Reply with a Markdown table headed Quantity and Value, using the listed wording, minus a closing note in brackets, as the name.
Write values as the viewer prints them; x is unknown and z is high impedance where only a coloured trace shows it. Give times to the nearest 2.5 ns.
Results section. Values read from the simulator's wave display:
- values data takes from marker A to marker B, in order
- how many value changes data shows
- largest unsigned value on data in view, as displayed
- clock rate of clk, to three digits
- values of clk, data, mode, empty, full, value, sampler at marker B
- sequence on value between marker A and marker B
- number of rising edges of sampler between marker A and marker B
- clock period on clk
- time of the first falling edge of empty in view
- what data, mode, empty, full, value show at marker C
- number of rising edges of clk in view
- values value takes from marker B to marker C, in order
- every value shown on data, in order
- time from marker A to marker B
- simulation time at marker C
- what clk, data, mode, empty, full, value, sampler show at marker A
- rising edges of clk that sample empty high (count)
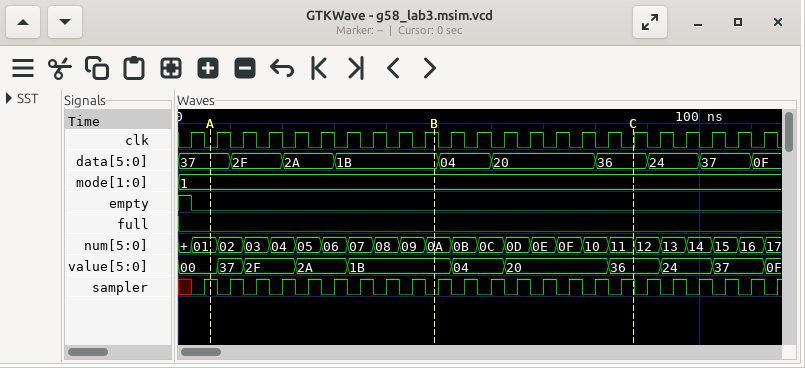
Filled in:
| Quantity | Value |
|---|---|
| values data takes from marker A to marker B, in order | 37, 2F, 2A, 1B |
| how many value changes data shows | 9 |
| largest unsigned value on data in view, as displayed | 37 |
| clock rate of clk, to three digits | 200 MHz |
| values of clk, data, mode, empty, full, value, sampler at marker B | clk=1, data=1B, mode=1, empty=0, full=0, value=1B, sampler=0 |
| sequence on value between marker A and marker B | 00, 37, 2F, 2A, 1B |
| number of rising edges of sampler between marker A and marker B | 8 |
| clock period on clk | 5 ns |
| time of the first falling edge of empty in view | 2.5 ns |
| what data, mode, empty, full, value show at marker C | data=36, mode=1, empty=0, full=0, value=36 |
| number of rising edges of clk in view | 23 |
| values value takes from marker B to marker C, in order | 1B, 04, 20, 36 |
| every value shown on data, in order | 37, 2F, 2A, 1B, 04, 20, 36, 24, 37, 0F |
| time from marker A to marker B | 42.5 ns |
| simulation time at marker C | 87.5 ns |
| what clk, data, mode, empty, full, value, sampler show at marker A | clk=0, data=37, mode=1, empty=0, full=0, value=00, sampler=1 |
| rising edges of clk that sample empty high | 1 |
